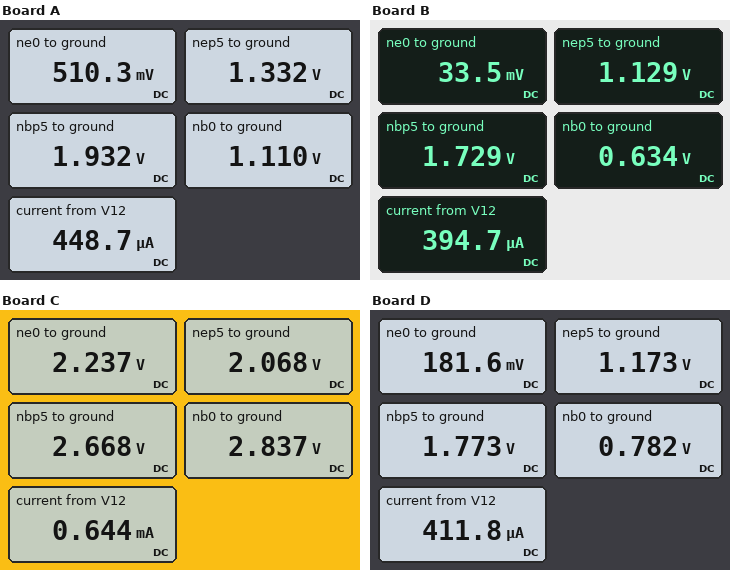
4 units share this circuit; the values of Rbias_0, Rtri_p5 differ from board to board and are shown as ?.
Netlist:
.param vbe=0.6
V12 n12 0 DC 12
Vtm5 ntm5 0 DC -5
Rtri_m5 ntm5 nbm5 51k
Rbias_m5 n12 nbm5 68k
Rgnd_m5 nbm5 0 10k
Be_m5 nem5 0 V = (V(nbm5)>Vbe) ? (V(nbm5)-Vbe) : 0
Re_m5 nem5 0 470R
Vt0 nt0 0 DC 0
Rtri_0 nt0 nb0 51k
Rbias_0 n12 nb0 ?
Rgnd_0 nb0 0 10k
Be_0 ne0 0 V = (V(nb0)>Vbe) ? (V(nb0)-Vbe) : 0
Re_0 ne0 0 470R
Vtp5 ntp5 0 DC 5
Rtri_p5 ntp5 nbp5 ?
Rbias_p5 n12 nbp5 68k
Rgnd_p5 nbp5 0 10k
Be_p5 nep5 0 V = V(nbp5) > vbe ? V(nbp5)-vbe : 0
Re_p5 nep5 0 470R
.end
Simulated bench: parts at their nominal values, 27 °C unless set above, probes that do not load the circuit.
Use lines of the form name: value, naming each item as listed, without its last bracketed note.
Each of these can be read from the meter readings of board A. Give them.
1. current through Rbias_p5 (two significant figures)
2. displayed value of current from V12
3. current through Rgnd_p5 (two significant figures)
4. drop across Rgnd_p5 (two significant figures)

current through Rbias_p5: 150 µA
displayed value of current from V12: 448.7 µA
current through Rgnd_p5: 190 µA
drop across Rgnd_p5: 1.9 V
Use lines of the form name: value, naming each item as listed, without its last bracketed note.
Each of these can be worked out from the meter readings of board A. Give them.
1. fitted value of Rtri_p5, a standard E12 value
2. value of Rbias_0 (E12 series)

fitted value of Rtri_p5, a standard E12 value: 68 kΩ
value of Rbias_0: 82 kΩ
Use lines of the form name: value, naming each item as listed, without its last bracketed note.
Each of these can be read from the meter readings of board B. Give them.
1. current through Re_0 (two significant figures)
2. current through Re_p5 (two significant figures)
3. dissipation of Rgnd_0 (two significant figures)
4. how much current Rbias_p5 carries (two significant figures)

current through Re_0: 71 µA
current through Re_p5: 2.4 mA
dissipation of Rgnd_0: 40 µW
how much current Rbias_p5 carries: 150 µA
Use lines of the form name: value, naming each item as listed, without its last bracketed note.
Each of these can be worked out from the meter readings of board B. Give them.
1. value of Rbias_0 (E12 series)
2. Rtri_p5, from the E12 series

value of Rbias_0: 150 kΩ
Rtri_p5, from the E12 series: 150 kΩ
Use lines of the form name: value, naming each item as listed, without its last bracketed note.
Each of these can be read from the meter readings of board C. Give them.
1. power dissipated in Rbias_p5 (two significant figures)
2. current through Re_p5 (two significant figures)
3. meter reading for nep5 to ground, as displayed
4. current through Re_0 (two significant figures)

power dissipated in Rbias_p5: 1.3 mW
current through Re_p5: 4.4 mA
meter reading for nep5 to ground, as displayed: 2.068 V
current through Re_0: 4.8 mA
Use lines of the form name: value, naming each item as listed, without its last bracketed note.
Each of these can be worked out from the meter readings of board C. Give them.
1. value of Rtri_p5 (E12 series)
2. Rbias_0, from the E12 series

value of Rtri_p5: 18 kΩ
Rbias_0, from the E12 series: 27 kΩ
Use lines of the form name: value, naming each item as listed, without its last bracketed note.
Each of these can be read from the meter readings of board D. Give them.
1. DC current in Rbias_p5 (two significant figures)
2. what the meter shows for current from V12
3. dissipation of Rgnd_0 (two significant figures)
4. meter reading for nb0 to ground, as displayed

DC current in Rbias_p5: 150 µA
what the meter shows for current from V12: 411.8 µA
dissipation of Rgnd_0: 61 µW
meter reading for nb0 to ground, as displayed: 0.782 V
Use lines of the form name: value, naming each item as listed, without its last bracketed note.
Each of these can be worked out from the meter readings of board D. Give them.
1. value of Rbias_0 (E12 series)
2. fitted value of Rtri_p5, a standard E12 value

value of Rbias_0: 120 kΩ
fitted value of Rtri_p5, a standard E12 value: 120 kΩ
